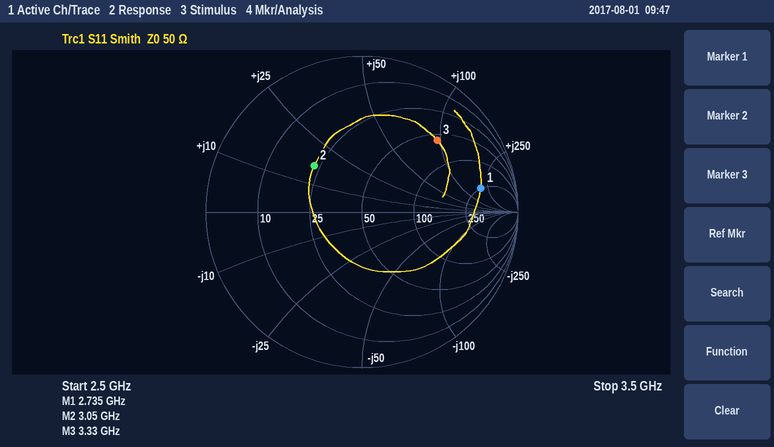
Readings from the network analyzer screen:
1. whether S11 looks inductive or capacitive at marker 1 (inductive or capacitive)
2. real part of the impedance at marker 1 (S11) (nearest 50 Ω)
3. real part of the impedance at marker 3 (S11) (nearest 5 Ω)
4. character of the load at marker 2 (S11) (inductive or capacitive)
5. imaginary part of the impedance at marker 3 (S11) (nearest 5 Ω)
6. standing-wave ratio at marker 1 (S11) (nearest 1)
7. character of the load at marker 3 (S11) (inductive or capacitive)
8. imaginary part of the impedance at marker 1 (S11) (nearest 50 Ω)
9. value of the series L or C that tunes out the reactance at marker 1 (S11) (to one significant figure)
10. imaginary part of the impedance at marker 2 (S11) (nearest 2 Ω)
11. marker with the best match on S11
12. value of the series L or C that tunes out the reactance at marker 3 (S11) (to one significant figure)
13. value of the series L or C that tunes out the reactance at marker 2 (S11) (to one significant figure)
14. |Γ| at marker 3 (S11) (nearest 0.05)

inductive
250 Ω
60 Ω
inductive
+95 Ω
8
inductive
+200 Ω
300 fF
+16 Ω
marker 2
500 fF
3 pF
0.65
